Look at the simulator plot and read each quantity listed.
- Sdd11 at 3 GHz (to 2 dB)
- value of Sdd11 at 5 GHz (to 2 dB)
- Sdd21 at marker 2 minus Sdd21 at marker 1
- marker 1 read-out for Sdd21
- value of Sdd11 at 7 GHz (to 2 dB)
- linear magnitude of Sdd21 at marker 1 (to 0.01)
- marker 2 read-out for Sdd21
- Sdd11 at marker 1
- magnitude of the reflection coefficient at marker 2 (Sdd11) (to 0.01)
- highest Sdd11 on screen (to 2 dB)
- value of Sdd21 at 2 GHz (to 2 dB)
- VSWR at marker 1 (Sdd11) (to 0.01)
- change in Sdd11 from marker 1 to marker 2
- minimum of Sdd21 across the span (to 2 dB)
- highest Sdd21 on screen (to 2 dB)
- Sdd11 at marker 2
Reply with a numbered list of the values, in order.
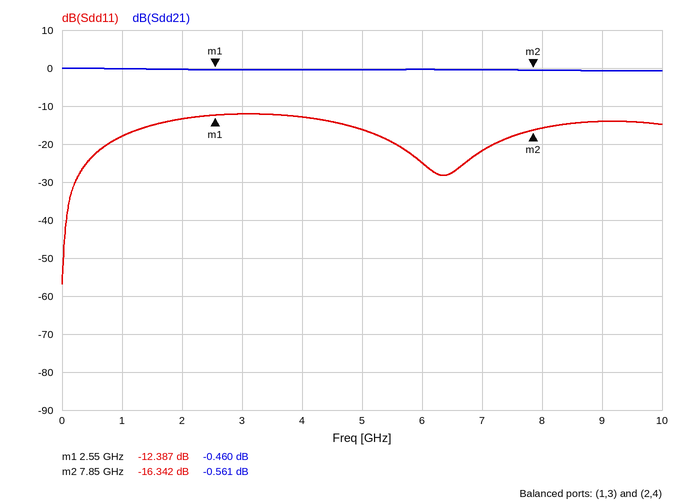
1. -12 dB
2. -16 dB
3. -0.101 dB
4. -0.460 dB
5. -22 dB
6. 0.95
7. -0.561 dB
8. -12.387 dB
9. 0.15
10. -12 dB
11. 0 dB
12. 1.63
13. -3.955 dB
14. 0 dB
15. 0 dB
16. -16.342 dB
